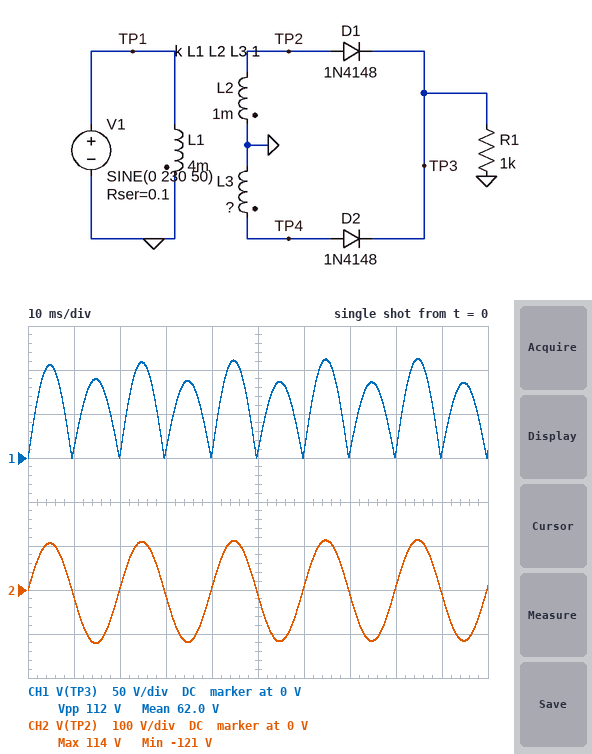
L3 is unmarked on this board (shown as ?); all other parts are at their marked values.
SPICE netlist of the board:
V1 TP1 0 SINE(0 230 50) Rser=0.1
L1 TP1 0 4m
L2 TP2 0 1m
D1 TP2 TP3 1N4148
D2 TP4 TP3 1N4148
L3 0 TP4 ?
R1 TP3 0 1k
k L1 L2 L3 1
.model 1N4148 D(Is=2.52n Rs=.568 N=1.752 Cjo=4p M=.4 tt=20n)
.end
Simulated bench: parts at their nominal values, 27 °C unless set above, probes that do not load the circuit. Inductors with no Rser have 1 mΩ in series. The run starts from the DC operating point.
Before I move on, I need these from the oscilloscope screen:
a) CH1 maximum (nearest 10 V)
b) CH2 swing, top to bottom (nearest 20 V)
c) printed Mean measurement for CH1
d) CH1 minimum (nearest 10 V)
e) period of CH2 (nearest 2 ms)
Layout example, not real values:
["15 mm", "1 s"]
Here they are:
["110 V", "240 V", "62.0 V", "0 V", "20 ms"]
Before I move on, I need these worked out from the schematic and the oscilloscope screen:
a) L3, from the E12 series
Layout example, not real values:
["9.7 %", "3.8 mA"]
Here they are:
["560 µH"]
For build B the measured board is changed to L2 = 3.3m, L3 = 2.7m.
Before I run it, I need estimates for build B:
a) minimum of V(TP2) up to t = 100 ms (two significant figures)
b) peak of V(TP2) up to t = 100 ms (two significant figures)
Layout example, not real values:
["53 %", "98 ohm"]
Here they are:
["-220 V", "210 V"]
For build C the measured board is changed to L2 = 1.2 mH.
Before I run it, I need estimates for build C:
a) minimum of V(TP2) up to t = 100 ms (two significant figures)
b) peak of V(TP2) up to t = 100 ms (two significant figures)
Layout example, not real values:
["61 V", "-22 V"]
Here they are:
["-130 V", "120 V"]
